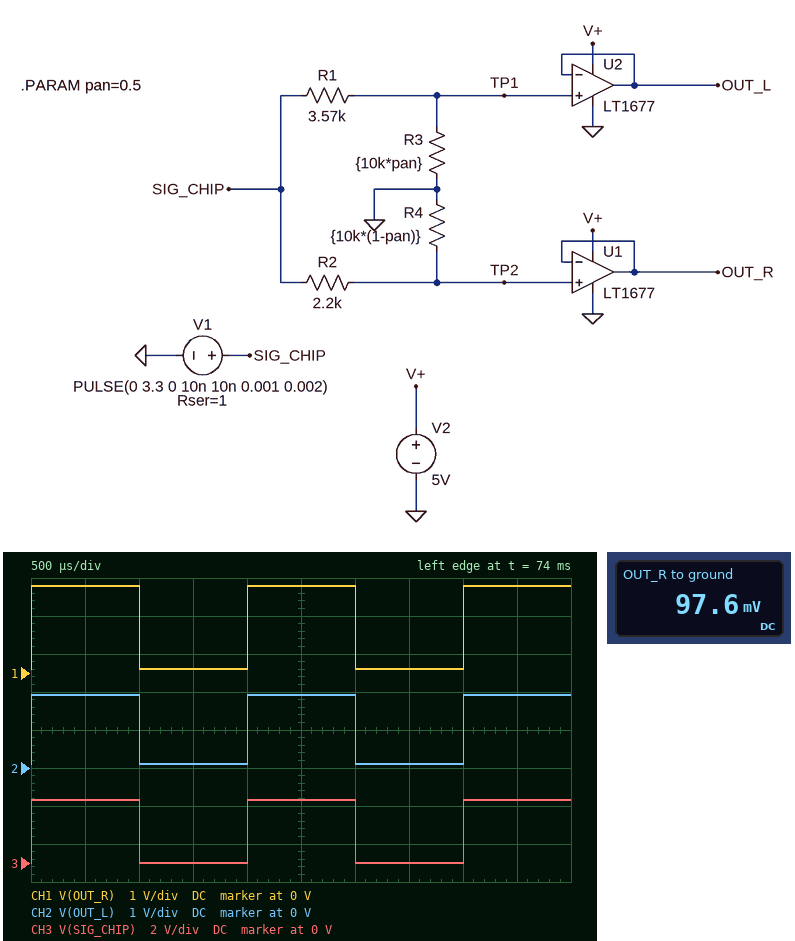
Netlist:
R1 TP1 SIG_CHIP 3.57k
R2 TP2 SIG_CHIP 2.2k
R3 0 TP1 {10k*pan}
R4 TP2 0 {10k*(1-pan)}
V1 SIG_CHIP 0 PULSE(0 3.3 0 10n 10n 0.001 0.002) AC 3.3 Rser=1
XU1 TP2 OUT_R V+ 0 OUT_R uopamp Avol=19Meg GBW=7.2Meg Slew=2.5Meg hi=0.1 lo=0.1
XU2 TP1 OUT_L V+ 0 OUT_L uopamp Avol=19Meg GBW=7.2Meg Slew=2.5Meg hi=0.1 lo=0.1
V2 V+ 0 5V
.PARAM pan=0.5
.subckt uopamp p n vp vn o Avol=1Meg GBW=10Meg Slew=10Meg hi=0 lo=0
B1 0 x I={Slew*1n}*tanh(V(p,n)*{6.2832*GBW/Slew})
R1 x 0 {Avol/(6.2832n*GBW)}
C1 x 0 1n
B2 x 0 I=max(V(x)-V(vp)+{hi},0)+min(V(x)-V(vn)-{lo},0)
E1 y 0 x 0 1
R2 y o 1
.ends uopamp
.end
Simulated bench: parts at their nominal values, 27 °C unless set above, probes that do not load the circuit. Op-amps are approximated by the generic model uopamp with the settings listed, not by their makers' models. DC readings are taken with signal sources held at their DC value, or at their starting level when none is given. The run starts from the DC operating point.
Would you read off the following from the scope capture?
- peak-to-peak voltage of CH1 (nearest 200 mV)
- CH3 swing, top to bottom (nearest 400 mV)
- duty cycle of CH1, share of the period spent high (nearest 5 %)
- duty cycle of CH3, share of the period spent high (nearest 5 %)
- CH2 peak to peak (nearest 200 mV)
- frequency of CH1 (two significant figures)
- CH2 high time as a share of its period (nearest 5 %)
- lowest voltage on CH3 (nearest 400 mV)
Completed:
2.2 V
3.2 V
50 %
50 %
1.8 V
500 Hz
50 %
0 V
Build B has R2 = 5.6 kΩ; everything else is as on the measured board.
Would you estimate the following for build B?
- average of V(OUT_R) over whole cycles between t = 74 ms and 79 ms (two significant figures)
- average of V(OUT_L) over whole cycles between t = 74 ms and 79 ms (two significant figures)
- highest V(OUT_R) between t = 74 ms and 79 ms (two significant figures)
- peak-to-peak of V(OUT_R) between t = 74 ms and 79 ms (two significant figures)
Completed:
830 mV
1.0 V
1.6 V
1.5 V
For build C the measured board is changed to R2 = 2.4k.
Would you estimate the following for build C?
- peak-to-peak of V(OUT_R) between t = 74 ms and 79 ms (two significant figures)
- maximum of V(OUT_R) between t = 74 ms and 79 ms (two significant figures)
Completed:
2.1 V
2.2 V
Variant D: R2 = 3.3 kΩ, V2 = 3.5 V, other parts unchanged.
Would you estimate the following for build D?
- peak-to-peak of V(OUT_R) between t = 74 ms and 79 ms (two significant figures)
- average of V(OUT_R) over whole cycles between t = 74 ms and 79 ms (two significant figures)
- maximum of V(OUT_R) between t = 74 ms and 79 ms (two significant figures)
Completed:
1.9 V
1.0 V
2.0 V
